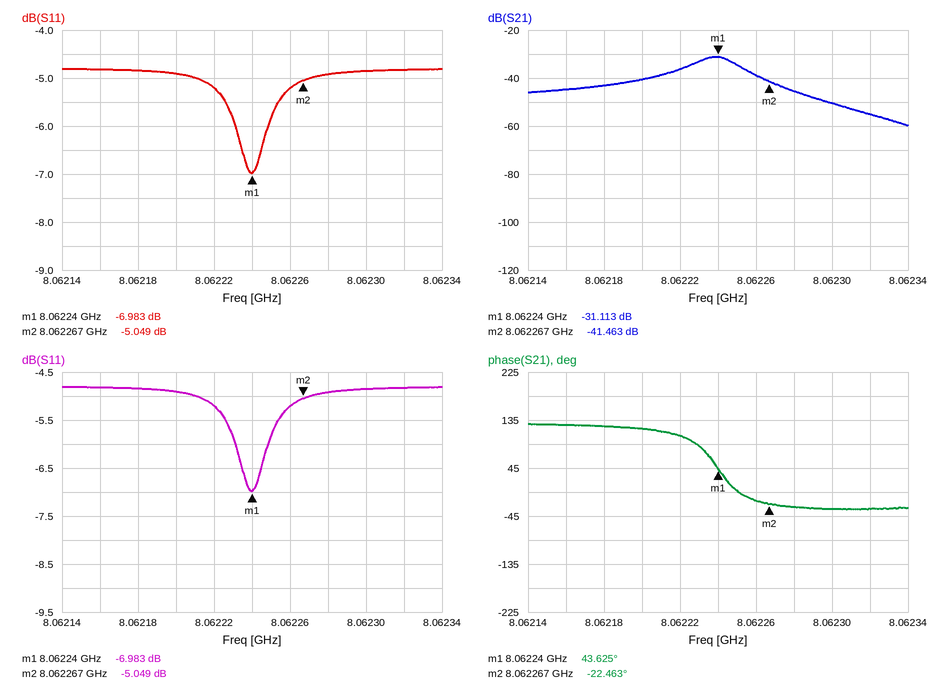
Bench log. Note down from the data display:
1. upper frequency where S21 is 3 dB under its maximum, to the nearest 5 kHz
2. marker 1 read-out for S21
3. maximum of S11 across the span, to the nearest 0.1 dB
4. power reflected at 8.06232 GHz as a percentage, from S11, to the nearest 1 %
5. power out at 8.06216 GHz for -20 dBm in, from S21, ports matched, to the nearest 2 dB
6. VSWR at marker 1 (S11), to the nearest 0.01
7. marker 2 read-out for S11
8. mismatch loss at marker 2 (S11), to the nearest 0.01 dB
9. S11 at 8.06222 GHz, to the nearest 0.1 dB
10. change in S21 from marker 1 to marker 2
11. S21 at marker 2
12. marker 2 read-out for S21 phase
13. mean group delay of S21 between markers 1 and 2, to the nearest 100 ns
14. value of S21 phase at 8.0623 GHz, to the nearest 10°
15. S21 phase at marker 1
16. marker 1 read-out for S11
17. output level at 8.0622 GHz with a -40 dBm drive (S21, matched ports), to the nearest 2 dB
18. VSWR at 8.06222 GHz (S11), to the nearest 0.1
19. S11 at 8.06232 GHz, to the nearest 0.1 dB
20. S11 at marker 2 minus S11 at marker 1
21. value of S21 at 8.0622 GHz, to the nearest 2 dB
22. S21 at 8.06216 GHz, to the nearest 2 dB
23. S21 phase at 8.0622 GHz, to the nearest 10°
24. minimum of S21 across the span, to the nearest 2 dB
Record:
8.062250 GHz
-31.113 dB
-4.8 dB
33 %
-64 dBm
2.62
-5.049 dB
1.63 dB
-5.2 dB
-10.350 dB
-41.463 dB
-22.463°
6.8 µs
-30°
43.625°
-6.983 dB
-80 dBm
3.4
-4.8 dB
1.934 dB
-40 dB
-44 dB
120°
-60 dB
